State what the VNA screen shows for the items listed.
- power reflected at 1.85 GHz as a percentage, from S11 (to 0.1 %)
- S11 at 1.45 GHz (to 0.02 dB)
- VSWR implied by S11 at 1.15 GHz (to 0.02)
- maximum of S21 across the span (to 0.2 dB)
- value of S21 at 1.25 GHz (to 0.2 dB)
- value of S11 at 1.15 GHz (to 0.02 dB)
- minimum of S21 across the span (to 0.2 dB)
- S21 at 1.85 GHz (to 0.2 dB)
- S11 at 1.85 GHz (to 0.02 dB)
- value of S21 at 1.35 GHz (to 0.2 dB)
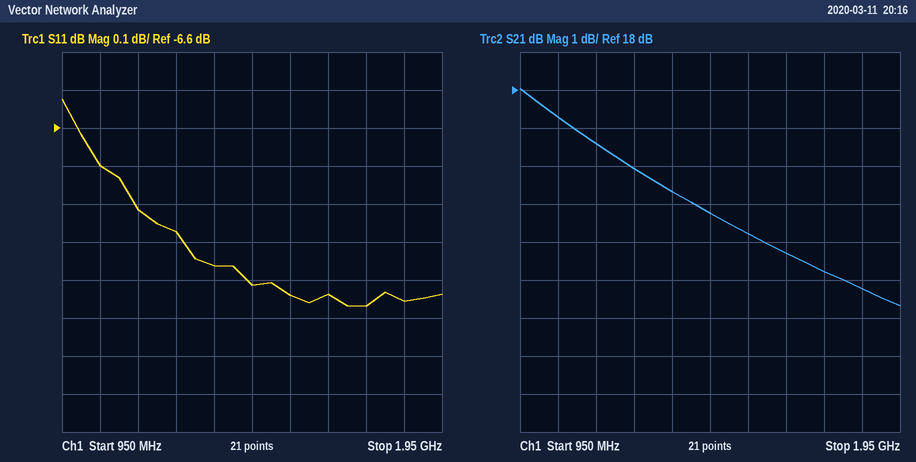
19.7 %
-7.02 dB
2.68
18.0 dB
16.0 dB
-6.82 dB
12.4 dB
12.8 dB
-7.06 dB
15.4 dB
